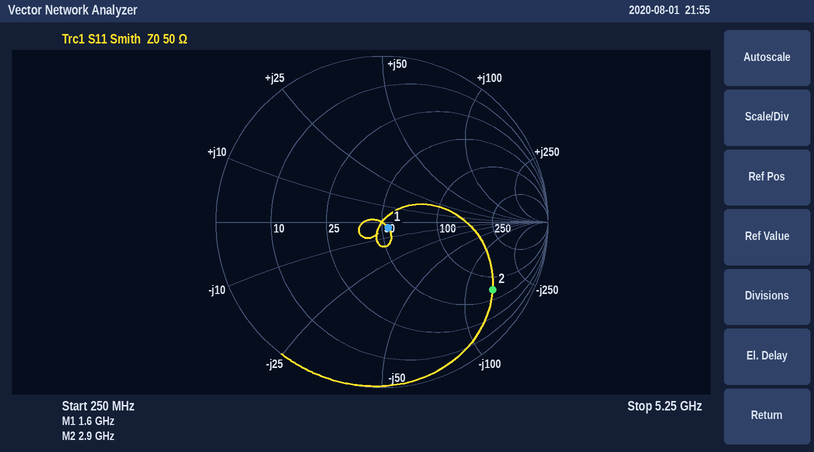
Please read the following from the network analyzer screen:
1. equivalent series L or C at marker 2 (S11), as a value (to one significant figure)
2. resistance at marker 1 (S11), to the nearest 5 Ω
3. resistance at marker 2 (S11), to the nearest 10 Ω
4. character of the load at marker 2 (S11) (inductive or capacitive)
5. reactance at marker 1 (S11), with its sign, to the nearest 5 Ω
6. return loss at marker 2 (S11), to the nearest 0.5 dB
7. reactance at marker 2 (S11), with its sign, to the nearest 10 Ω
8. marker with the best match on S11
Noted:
400 fF
55 Ω
70 Ω
capacitive
-5 Ω
2.0 dB
-150 Ω
marker 1
